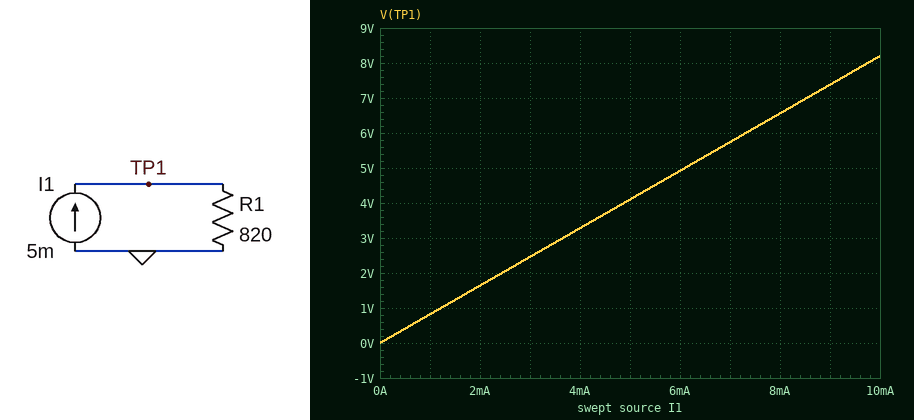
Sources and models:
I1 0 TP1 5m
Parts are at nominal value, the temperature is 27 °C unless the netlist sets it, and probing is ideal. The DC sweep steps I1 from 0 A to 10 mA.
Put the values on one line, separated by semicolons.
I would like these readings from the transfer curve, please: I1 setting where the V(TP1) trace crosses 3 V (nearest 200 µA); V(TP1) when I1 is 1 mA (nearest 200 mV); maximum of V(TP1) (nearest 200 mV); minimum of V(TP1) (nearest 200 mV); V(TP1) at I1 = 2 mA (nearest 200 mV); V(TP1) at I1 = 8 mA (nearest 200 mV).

3.6 mA; 800 mV; 8.2 V; 0 V; 1.6 V; 6.6 V
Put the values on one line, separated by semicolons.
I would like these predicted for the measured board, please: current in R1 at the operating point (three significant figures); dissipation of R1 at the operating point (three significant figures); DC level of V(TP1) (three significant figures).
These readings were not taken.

5.00 mA; 20.5 mW; 4.10 V
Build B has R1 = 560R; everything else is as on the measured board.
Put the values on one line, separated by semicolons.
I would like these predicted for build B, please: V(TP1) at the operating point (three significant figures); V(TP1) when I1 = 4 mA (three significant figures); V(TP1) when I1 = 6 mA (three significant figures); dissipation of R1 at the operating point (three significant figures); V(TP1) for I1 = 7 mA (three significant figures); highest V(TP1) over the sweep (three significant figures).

2.80 V; 2.24 V; 3.36 V; 14.0 mW; 3.92 V; 5.60 V
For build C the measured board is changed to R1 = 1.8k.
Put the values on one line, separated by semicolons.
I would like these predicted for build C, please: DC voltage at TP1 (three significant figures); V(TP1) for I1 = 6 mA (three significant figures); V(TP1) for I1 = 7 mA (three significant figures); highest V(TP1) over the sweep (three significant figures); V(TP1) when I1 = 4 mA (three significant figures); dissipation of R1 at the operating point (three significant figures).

9.00 V; 10.8 V; 12.6 V; 18.0 V; 7.20 V; 45.0 mW
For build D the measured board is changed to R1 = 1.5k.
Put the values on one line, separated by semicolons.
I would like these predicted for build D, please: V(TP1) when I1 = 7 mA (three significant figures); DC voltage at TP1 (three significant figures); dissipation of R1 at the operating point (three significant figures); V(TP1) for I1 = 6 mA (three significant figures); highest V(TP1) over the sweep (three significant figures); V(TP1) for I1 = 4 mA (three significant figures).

10.5 V; 7.50 V; 37.5 mW; 9.00 V; 15.0 V; 6.00 V
